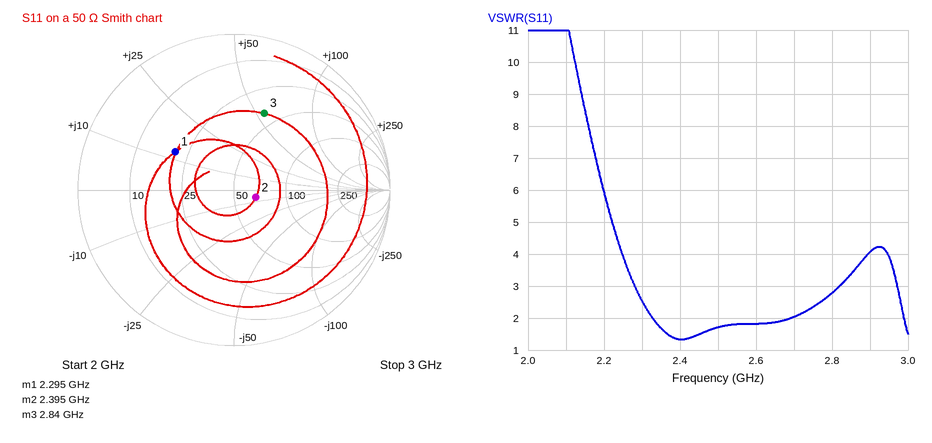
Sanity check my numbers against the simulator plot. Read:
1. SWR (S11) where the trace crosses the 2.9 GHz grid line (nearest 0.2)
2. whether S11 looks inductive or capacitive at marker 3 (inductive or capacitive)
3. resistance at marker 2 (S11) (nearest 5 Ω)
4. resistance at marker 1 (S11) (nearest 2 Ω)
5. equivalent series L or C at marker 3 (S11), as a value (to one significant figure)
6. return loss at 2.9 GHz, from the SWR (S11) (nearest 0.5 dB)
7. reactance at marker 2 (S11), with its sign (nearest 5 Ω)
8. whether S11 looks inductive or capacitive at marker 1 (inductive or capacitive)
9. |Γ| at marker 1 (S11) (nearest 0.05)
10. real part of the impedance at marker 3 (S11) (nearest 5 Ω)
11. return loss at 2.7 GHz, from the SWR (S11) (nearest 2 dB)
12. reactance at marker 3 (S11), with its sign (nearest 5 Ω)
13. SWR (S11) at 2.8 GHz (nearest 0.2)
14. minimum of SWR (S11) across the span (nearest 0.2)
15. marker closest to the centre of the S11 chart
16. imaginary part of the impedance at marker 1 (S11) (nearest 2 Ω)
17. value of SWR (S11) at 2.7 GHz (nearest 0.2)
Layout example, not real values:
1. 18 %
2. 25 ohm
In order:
1. 4.0
2. inductive
3. 65 Ω
4. 20 Ω
5. 3 nH
6. 4.5 dB
7. -5 Ω
8. inductive
9. 0.45
10. 40 Ω
11. 10 dB
12. +55 Ω
13. 2.8
14. 1.4
15. marker 2
16. +12 Ω
17. 2.0
